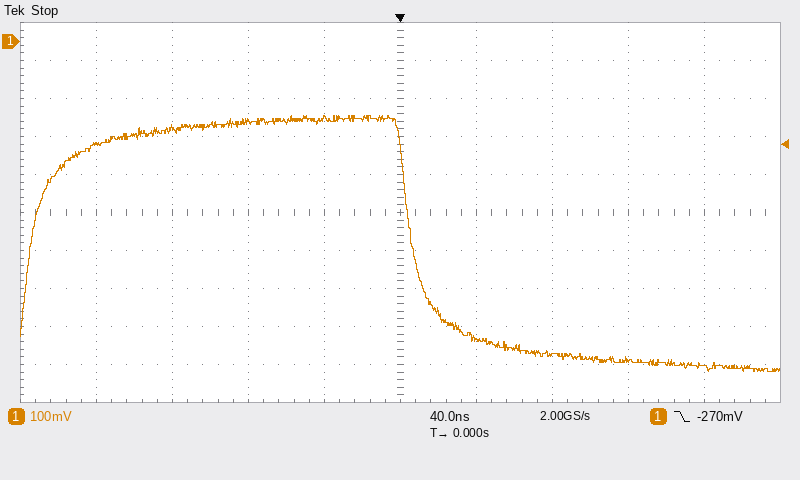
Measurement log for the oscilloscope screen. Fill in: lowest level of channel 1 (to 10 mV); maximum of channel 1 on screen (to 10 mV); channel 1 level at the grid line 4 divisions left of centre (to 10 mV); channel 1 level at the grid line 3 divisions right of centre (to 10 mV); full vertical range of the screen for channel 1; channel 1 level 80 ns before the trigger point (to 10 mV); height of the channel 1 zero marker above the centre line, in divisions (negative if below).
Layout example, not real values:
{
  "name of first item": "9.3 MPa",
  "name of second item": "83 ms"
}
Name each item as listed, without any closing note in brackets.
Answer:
{
  "lowest level of channel 1": "-870 mV",
  "maximum of channel 1 on screen": "-190 mV",
  "channel 1 level at the grid line 4 divisions left of centre": "-270 mV",
  "channel 1 level at the grid line 3 divisions right of centre": "-840 mV",
  "full vertical range of the screen for channel 1": "1 V",
  "channel 1 level 80 ns before the trigger point": "-210 mV",
  "height of the channel 1 zero marker above the centre line, in divisions": "+4.5 div"
}
